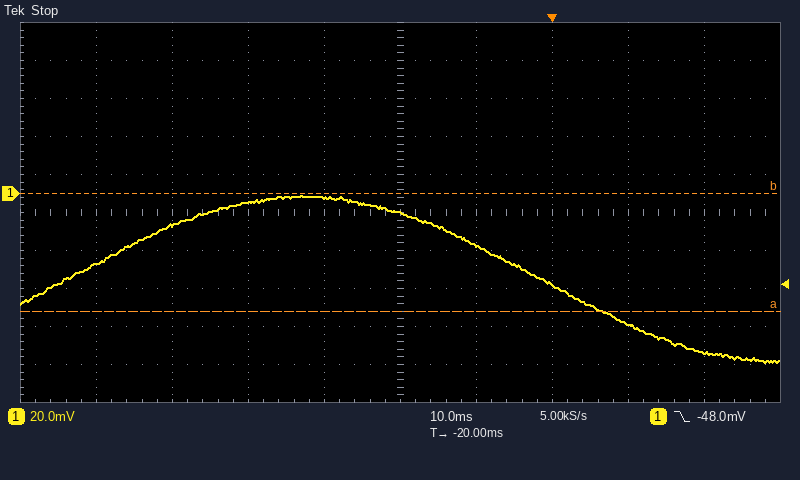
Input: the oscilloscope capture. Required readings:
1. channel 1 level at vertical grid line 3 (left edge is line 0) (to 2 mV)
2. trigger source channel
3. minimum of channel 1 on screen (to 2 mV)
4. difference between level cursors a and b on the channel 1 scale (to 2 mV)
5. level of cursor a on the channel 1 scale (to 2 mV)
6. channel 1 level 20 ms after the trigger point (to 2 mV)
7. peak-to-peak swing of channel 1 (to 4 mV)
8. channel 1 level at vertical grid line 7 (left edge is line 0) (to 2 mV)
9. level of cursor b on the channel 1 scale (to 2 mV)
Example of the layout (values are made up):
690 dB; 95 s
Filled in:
-4 mV; channel 1; -88 mV; 62 mV; -62 mV; -84 mV; 88 mV; -48 mV; 0 mV
